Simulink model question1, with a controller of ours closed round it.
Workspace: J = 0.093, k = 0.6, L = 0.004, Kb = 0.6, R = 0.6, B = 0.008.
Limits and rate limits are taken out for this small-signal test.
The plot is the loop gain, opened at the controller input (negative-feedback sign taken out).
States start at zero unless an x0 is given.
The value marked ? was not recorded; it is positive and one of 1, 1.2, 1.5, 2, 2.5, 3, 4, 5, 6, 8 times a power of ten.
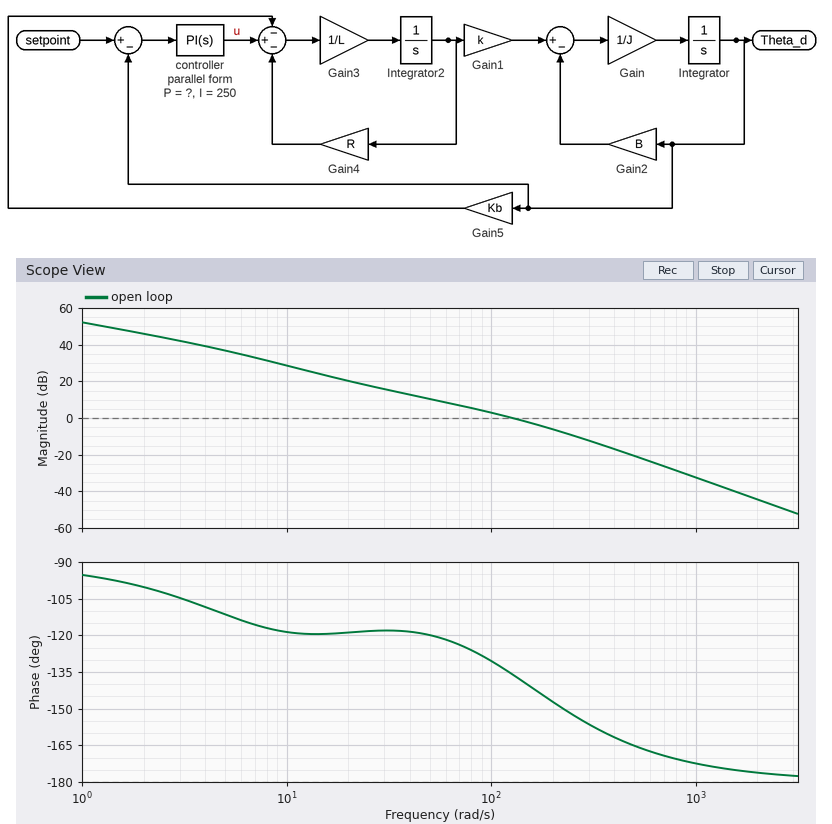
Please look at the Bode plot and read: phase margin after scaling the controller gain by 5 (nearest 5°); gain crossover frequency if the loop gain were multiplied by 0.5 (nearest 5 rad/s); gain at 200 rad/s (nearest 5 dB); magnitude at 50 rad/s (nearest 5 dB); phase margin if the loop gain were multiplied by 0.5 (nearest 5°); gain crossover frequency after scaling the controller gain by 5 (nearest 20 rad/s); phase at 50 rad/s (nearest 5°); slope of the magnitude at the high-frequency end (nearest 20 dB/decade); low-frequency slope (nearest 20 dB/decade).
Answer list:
20°
75 rad/s
-5 dB
10 dB
55°
340 rad/s
-120°
-40 dB/decade
-20 dB/decade
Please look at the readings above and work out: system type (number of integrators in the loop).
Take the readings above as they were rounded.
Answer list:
1
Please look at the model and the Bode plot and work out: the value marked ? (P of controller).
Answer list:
15
